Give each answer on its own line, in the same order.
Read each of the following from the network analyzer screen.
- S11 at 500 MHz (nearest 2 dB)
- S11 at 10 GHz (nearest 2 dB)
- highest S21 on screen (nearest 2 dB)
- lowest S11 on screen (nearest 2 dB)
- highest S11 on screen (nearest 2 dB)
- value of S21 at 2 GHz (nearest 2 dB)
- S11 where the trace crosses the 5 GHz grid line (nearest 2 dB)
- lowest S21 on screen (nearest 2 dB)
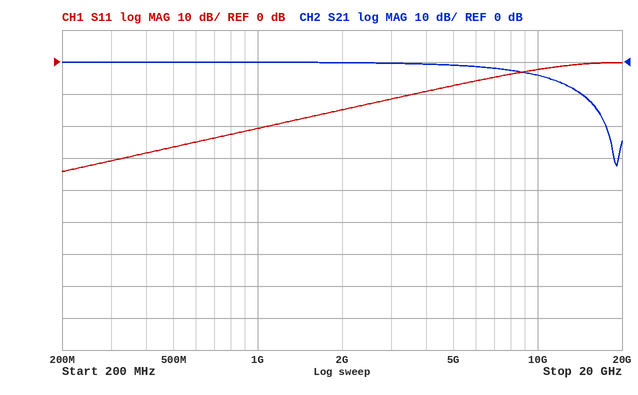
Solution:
-26 dB
-2 dB
0 dB
-34 dB
0 dB
0 dB
-8 dB
-32 dB
